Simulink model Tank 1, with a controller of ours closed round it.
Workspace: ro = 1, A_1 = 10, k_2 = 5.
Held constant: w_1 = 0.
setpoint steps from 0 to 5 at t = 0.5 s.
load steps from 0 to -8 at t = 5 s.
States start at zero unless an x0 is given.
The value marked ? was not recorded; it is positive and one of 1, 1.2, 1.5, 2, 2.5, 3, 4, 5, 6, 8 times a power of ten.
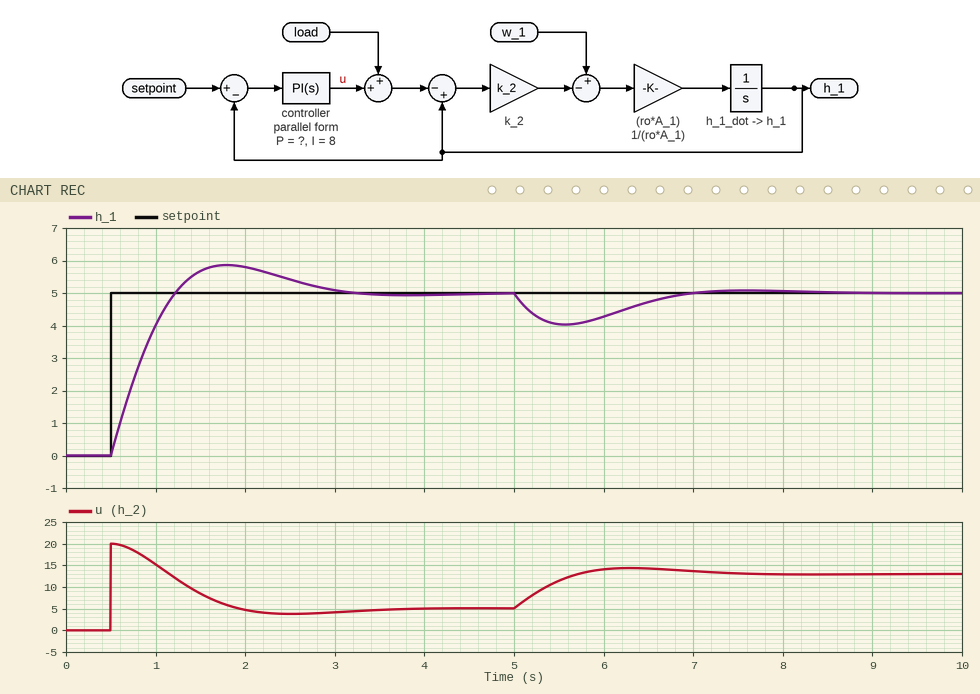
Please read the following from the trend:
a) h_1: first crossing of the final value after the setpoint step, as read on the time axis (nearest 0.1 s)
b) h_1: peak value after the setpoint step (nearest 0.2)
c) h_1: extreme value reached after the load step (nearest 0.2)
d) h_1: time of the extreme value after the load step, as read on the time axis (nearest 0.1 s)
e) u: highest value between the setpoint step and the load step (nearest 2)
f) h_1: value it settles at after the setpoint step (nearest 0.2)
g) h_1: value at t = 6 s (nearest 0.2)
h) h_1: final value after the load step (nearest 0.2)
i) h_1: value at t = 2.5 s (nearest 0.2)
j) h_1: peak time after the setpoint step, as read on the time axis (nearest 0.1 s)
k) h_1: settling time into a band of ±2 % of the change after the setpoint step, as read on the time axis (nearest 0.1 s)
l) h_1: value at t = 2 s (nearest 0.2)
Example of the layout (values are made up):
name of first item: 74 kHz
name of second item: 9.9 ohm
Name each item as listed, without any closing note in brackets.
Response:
h_1: first crossing of the final value after the setpoint step, as read on the time axis: 1.2 s
h_1: peak value after the setpoint step: 5.8
h_1: extreme value reached after the load step: 4.0
h_1: time of the extreme value after the load step, as read on the time axis: 5.6 s
u: highest value between the setpoint step and the load step: 20
h_1: value it settles at after the setpoint step: 5.0
h_1: value at t = 6 s: 4.2
h_1: final value after the load step: 5.0
h_1: value at t = 2.5 s: 5.4
h_1: peak time after the setpoint step, as read on the time axis: 1.8 s
h_1: settling time into a band of ±2 % of the change after the setpoint step, as read on the time axis: 3.0 s
h_1: value at t = 2 s: 5.8
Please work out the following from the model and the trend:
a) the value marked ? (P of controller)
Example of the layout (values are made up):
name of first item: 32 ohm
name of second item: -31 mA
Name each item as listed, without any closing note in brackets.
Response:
the value marked ?: 4
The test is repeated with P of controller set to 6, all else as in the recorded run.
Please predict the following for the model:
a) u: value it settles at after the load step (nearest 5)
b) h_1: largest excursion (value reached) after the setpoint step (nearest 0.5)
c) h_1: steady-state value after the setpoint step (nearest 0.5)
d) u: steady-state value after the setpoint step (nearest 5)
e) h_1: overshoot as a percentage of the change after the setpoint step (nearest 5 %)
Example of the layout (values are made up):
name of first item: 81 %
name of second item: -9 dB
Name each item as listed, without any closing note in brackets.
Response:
u: value it settles at after the load step: 15
h_1: largest excursion (value reached) after the setpoint step: 5.5
h_1: steady-state value after the setpoint step: 5.0
u: steady-state value after the setpoint step: 5
h_1: overshoot as a percentage of the change after the setpoint step: 10 %
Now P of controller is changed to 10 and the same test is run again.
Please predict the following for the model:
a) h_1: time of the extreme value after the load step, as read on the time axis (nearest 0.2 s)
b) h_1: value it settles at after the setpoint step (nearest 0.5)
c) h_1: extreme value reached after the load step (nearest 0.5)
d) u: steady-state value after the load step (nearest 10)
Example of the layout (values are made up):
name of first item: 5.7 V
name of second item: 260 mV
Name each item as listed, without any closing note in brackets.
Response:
h_1: time of the extreme value after the load step, as read on the time axis: 5.4 s
h_1: value it settles at after the setpoint step: 5.0
h_1: extreme value reached after the load step: 4.5
u: steady-state value after the load step: 10
